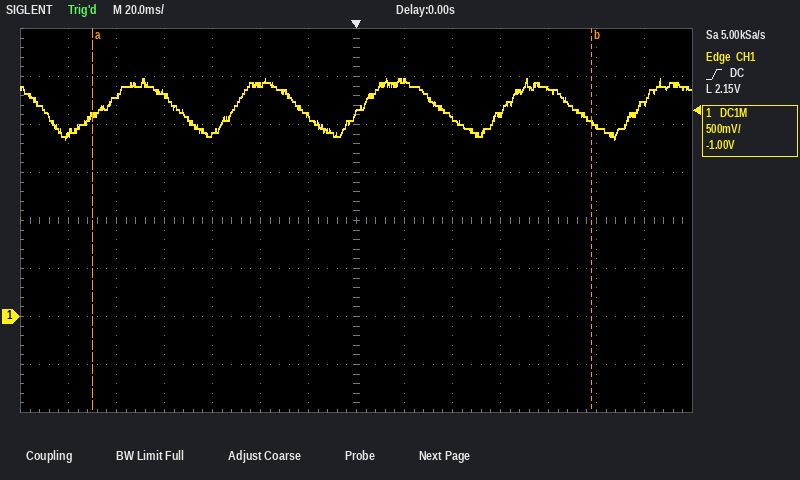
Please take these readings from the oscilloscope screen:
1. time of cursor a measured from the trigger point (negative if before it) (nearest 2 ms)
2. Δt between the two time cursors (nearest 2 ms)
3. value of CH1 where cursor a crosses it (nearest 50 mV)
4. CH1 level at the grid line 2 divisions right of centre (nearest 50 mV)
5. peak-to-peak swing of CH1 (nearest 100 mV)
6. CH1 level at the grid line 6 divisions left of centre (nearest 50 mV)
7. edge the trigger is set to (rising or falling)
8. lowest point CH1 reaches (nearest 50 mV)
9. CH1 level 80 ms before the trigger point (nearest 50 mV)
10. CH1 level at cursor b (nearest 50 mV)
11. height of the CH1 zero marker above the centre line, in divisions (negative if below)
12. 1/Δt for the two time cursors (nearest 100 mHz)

-110 ms
208 ms
2.10 V
2.05 V
600 mV
1.90 V
rising
1.85 V
2.30 V
2.00 V
-2.0 div
4.8 Hz
